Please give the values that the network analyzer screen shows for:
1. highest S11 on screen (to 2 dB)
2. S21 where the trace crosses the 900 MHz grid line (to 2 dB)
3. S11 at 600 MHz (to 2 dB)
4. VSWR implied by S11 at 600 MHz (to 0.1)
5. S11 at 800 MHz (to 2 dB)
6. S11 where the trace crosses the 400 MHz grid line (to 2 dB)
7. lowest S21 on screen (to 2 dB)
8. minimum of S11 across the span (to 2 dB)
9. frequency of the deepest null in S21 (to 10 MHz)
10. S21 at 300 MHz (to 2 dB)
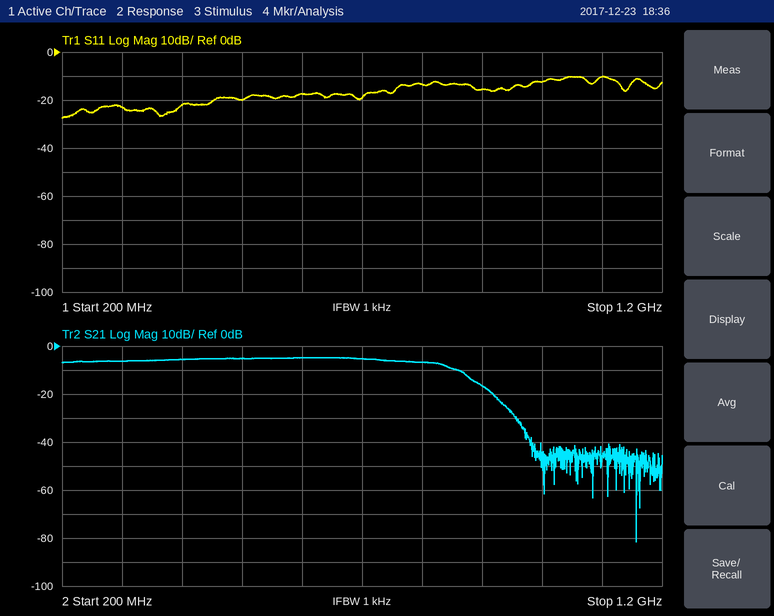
-10 dB
-16 dB
-18 dB
1.3
-14 dB
-22 dB
-82 dB
-28 dB
1.16 GHz
-6 dB
